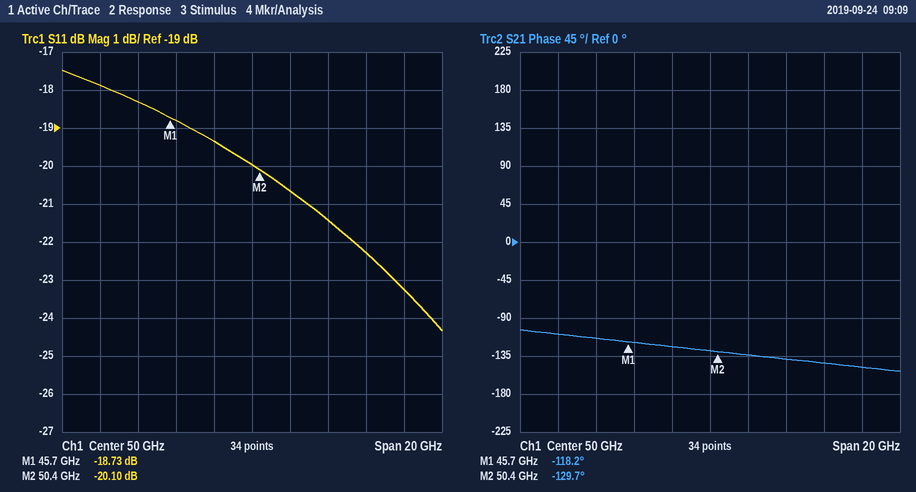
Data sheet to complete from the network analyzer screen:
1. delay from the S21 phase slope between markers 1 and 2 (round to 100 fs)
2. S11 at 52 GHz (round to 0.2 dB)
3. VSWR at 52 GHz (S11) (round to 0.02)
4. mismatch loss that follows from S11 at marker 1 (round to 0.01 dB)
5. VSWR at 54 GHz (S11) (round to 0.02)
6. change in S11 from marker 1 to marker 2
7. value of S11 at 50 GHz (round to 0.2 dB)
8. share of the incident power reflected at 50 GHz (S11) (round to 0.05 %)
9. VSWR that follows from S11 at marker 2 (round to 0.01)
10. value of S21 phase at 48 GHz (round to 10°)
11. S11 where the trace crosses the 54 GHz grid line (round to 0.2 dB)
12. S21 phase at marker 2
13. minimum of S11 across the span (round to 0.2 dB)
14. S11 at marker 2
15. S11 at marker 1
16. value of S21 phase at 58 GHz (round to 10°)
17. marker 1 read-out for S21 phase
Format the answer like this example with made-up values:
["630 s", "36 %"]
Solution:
["6.8 ps", "-20.6 dB", "1.20", "0.06 dB", "1.18", "-1.37 dB", "-20.0 dB", "1.00 %", "1.22", "-120°", "-21.4 dB", "-129.7°", "-24.4 dB", "-20.10 dB", "-18.73 dB", "-150°", "-118.2°"]
